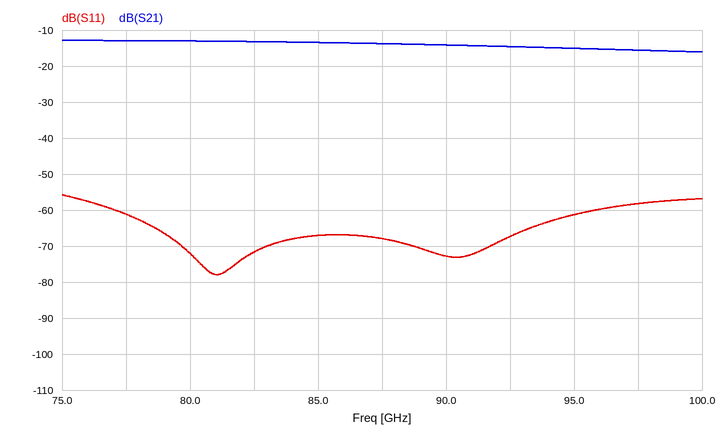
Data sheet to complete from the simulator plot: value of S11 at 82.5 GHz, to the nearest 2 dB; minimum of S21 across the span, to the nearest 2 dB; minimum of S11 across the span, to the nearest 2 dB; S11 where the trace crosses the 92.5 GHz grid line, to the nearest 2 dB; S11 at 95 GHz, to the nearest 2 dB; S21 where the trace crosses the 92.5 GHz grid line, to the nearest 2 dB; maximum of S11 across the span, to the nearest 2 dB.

-72 dB
-16 dB
-78 dB
-68 dB
-62 dB
-14 dB
-56 dB
